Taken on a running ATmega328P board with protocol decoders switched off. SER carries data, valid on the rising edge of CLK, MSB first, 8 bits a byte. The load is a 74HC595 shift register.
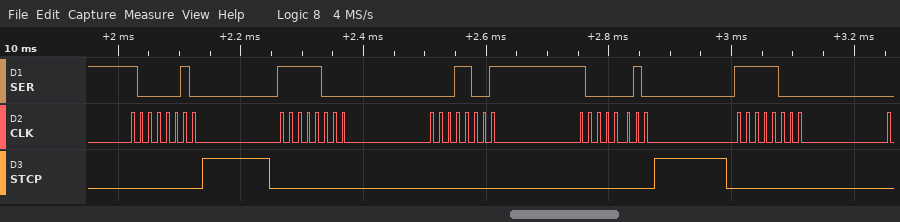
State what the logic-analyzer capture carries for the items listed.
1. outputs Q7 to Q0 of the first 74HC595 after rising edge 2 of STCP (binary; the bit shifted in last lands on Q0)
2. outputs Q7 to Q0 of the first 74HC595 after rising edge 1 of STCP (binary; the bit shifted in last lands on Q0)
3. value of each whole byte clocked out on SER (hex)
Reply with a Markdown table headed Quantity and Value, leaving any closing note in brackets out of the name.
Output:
| Quantity | Value |
|---|---|
| outputs Q7 to Q0 of the first 74HC595 after rising edge 2 of STCP | 10000010 |
| outputs Q7 to Q0 of the first 74HC595 after rising edge 1 of STCP | 10000010 |
| value of each whole byte clocked out on SER | 82 F8 19 82 F8 |
